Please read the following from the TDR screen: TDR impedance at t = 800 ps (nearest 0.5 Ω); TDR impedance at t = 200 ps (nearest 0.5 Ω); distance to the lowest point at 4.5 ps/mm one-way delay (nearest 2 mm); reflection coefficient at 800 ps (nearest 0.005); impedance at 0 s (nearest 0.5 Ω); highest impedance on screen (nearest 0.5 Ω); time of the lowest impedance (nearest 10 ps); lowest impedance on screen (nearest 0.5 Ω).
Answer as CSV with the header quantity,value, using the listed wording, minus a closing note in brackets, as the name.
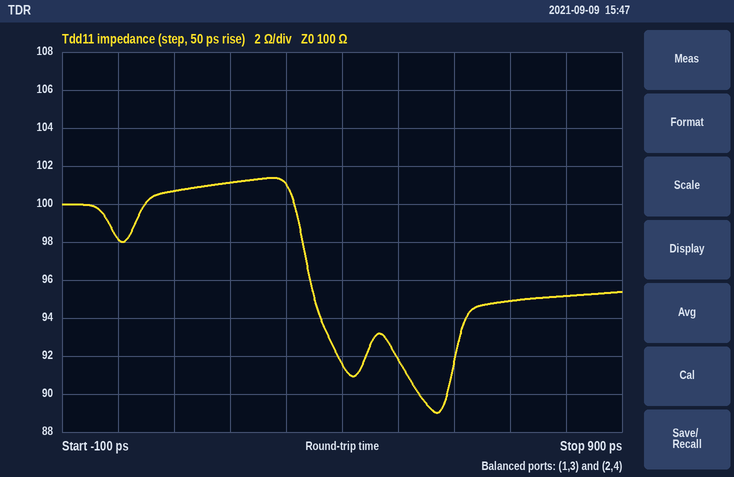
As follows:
quantity,value
TDR impedance at t = 800 ps,95.0 Ω
TDR impedance at t = 200 ps,101.0 Ω
distance to the lowest point at 4.5 ps/mm one-way delay,64 mm
reflection coefficient at 800 ps,-0.025
impedance at 0 s,98.0 Ω
highest impedance on screen,101.5 Ω
time of the lowest impedance,570 ps
lowest impedance on screen,89.0 Ω
